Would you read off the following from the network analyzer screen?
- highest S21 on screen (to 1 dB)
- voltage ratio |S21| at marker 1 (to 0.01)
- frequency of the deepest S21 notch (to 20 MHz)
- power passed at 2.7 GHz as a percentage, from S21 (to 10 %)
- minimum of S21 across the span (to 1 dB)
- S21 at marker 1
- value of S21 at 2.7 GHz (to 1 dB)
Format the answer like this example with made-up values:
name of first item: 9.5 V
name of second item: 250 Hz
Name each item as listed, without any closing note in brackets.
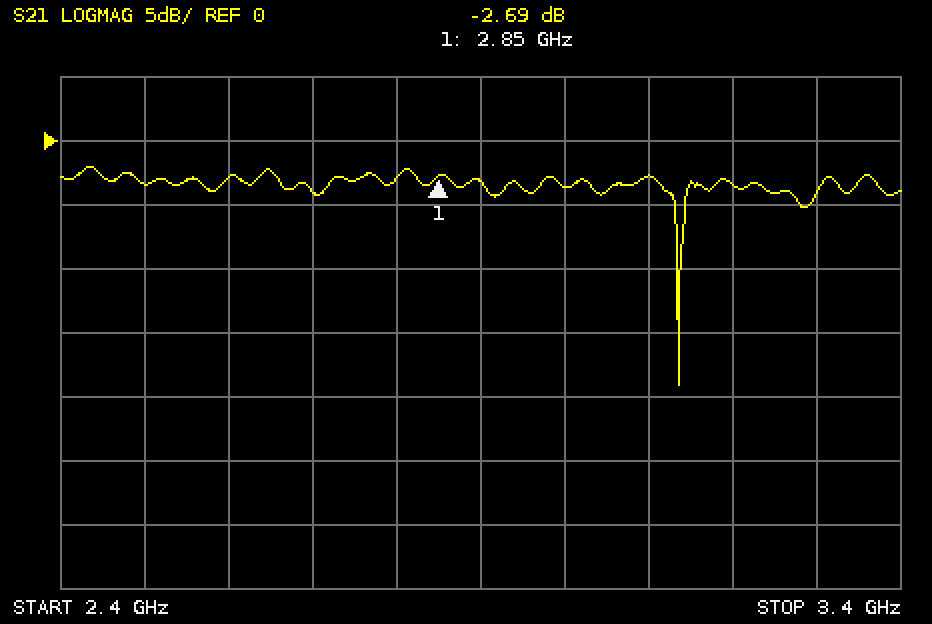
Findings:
highest S21 on screen: -2 dB
voltage ratio |S21| at marker 1: 0.73
frequency of the deepest S21 notch: 3.14 GHz
power passed at 2.7 GHz as a percentage, from S21: 40 %
minimum of S21 across the span: -19 dB
S21 at marker 1: -2.69 dB
value of S21 at 2.7 GHz: -4 dB
